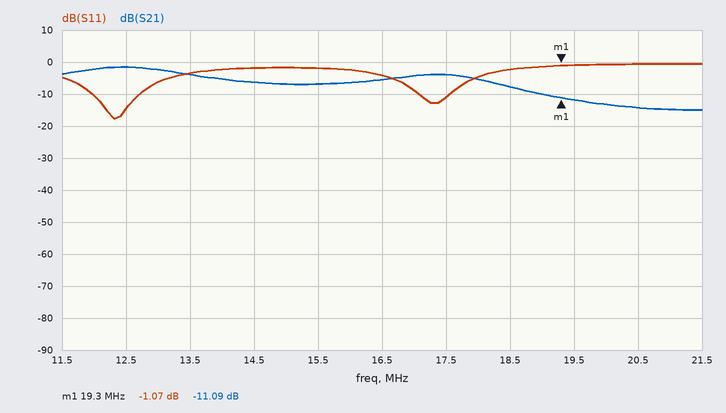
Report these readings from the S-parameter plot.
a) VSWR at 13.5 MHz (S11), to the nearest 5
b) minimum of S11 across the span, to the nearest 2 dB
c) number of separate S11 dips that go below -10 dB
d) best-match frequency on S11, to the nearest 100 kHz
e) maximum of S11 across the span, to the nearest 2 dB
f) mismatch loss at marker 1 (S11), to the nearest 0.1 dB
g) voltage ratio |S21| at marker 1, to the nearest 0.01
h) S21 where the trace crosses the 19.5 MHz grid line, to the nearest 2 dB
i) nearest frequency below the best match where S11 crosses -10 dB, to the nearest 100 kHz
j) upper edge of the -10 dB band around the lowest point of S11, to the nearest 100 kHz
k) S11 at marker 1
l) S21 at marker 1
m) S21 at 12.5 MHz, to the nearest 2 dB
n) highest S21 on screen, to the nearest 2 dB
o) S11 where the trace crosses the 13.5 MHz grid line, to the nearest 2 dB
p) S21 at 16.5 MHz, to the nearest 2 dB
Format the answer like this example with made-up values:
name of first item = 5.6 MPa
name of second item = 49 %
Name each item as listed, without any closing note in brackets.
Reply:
VSWR at 13.5 MHz (S11), to the nearest 5 = 5
minimum of S11 across the span, to the nearest 2 dB = -18 dB
number of separate S11 dips that go below -10 dB = 2
best-match frequency on S11, to the nearest 100 kHz = 12.3 MHz
maximum of S11 across the span, to the nearest 2 dB = 0 dB
mismatch loss at marker 1 (S11), to the nearest 0.1 dB = 6.6 dB
voltage ratio |S21| at marker 1, to the nearest 0.01 = 0.28
S21 where the trace crosses the 19.5 MHz grid line, to the nearest 2 dB = -12 dB
nearest frequency below the best match where S11 crosses -10 dB, to the nearest 100 kHz = 12.0 MHz
upper edge of the -10 dB band around the lowest point of S11, to the nearest 100 kHz = 12.7 MHz
S11 at marker 1 = -1.07 dB
S21 at marker 1 = -11.09 dB
S21 at 12.5 MHz, to the nearest 2 dB = -2 dB
highest S21 on screen, to the nearest 2 dB = -2 dB
S11 where the trace crosses the 13.5 MHz grid line, to the nearest 2 dB = -4 dB
S21 at 16.5 MHz, to the nearest 2 dB = -6 dB
